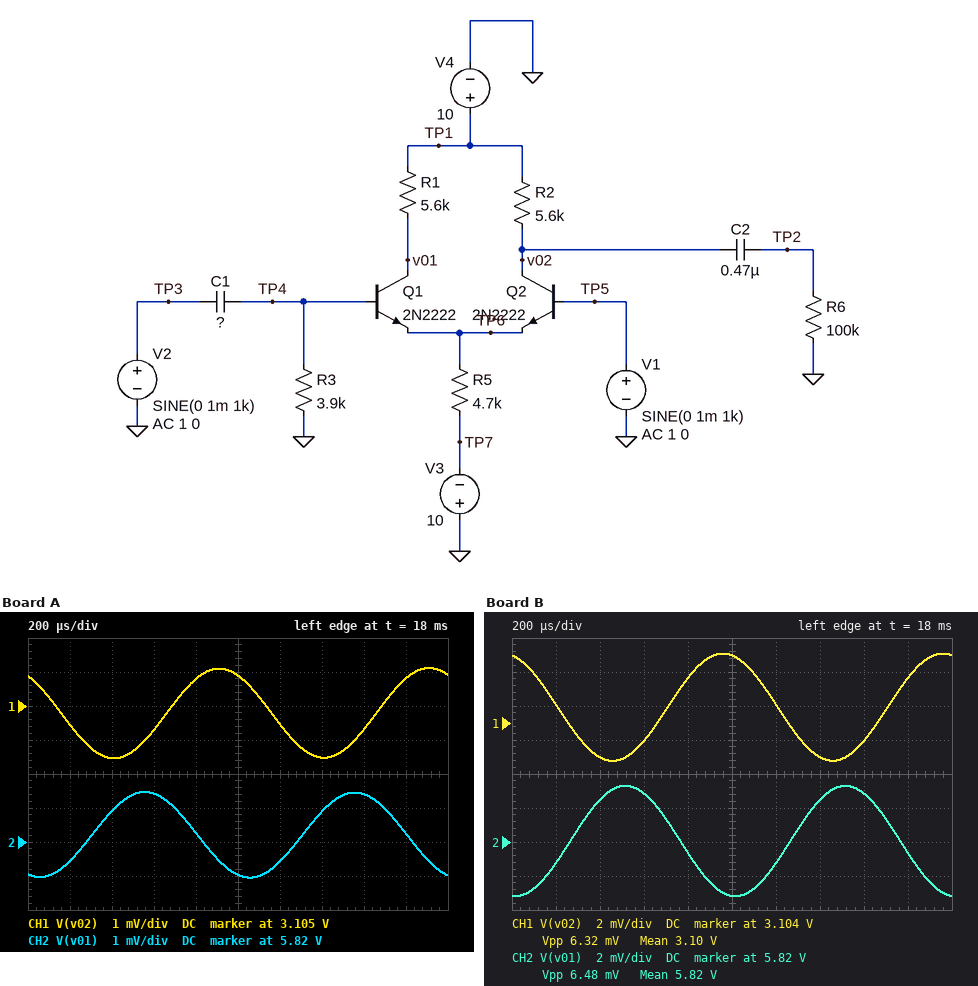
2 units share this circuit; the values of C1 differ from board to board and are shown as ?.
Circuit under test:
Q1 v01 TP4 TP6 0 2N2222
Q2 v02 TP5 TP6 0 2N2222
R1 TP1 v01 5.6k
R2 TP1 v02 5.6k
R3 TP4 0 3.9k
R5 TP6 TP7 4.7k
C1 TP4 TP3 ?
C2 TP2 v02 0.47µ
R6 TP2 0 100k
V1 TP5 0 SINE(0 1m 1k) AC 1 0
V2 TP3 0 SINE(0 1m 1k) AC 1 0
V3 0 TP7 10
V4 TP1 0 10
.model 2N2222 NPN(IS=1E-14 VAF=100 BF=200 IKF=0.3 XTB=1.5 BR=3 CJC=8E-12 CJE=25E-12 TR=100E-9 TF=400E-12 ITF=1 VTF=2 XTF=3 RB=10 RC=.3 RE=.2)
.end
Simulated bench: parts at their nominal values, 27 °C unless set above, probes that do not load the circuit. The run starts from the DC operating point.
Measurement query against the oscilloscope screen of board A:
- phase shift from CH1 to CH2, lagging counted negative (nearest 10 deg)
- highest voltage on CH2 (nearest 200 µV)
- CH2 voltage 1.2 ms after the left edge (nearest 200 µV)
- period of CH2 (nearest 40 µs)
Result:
130 deg
5.8214 V
5.8194 V
1.00 ms
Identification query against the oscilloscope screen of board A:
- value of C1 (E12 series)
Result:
3.3 µF
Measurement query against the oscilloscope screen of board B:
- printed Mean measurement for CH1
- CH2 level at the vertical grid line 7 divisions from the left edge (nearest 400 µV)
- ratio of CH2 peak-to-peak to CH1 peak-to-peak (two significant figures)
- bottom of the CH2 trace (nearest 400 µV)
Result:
3.10 V
5.8224 V
1.0
5.8168 V
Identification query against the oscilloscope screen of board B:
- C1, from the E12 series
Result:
1.2 µF
